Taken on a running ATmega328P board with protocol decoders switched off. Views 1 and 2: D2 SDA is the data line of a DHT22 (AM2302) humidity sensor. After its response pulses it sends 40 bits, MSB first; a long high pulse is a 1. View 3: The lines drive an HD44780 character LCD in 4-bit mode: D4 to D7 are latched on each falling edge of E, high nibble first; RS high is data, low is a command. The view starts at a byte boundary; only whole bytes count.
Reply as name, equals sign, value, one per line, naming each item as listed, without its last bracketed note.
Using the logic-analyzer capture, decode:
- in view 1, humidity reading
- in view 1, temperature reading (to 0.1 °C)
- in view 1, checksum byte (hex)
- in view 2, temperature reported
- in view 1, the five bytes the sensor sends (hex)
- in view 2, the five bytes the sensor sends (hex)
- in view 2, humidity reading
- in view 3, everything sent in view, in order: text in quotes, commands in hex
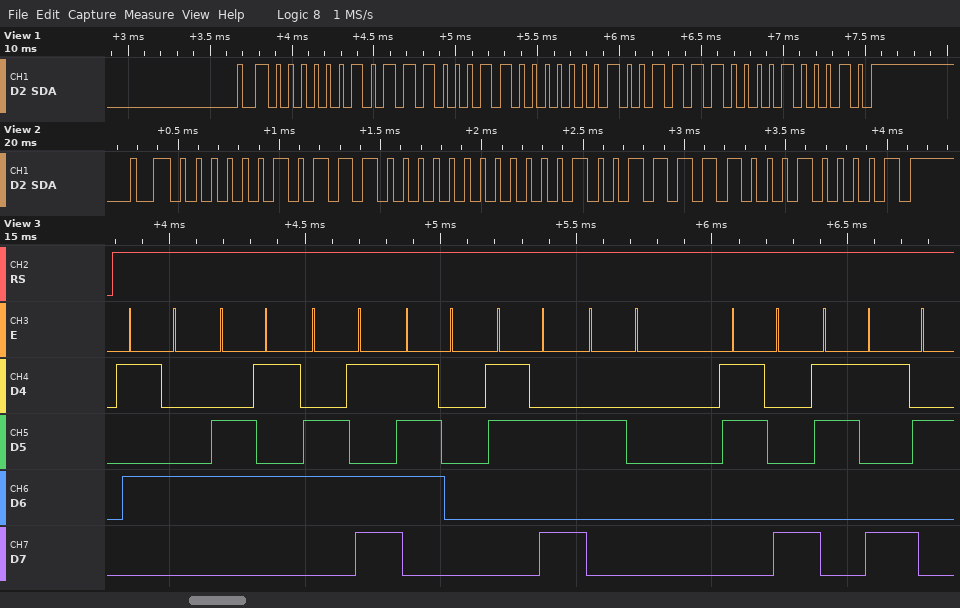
in view 1, humidity reading = 73.9 %
in view 1, temperature reading = 31.6 °C
in view 1, checksum byte = 0x22
in view 2, temperature reported = 31.8 °C
in view 1, the five bytes the sensor sends = 02 E3 01 3C 22
in view 2, the five bytes the sensor sends = 02 E0 01 3E 21
in view 2, humidity reading = 73.6 %
in view 3, everything sent in view, in order: text in quotes, commands in hex = "Temp: 89"
